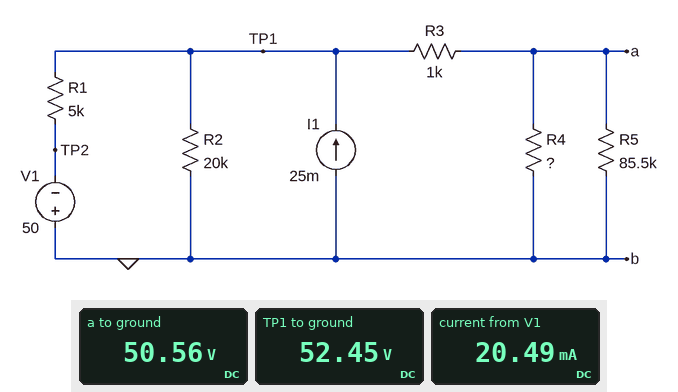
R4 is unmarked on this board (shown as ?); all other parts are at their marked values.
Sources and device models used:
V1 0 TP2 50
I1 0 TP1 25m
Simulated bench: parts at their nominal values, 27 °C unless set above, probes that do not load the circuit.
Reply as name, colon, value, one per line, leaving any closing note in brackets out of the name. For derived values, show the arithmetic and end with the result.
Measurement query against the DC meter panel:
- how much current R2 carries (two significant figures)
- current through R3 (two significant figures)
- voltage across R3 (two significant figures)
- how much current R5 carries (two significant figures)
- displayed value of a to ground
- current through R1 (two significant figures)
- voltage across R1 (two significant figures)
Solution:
how much current R2 carries: (52.45 V) / 20 kΩ = 2.6 mA
current through R3: (52.45 V - 50.56 V) / 1 kΩ = 1.9 mA
voltage across R3: 52.45 V - 50.56 V = 1.9 V
how much current R5 carries: (50.56 V) / 85.5 kΩ = 590 µA
displayed value of a to ground: 50.56 V
current through R1: (52.45 V - (-50 V)) / 5 kΩ = 20 mA
voltage across R1: 52.45 V - (-50 V) = 100 V
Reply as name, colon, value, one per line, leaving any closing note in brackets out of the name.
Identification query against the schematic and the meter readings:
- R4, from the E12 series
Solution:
R4, from the E12 series: 39 kΩ
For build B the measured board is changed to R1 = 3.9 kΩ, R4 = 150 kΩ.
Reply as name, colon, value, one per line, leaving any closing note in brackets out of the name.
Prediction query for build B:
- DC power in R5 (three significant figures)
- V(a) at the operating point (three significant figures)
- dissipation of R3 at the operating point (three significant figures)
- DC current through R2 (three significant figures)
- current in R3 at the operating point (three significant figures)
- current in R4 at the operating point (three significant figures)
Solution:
DC power in R5: 15.9 mW
V(a) at the operating point: 36.9 V
dissipation of R3 at the operating point: 458 µW
DC current through R2: 1.88 mA
current in R3 at the operating point: 677 µA
current in R4 at the operating point: 246 µA
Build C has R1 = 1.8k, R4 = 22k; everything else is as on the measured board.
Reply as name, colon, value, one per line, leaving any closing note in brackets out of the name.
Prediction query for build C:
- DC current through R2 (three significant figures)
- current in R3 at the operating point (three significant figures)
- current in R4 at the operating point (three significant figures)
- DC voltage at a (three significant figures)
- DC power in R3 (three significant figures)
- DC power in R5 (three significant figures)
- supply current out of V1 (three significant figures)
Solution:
DC current through R2: 211 µA
current in R3 at the operating point: 228 µA
current in R4 at the operating point: 181 µA
DC voltage at a: -3.98 V
DC power in R3: 51.8 µW
DC power in R5: 186 µW
supply current out of V1: 25.4 mA
